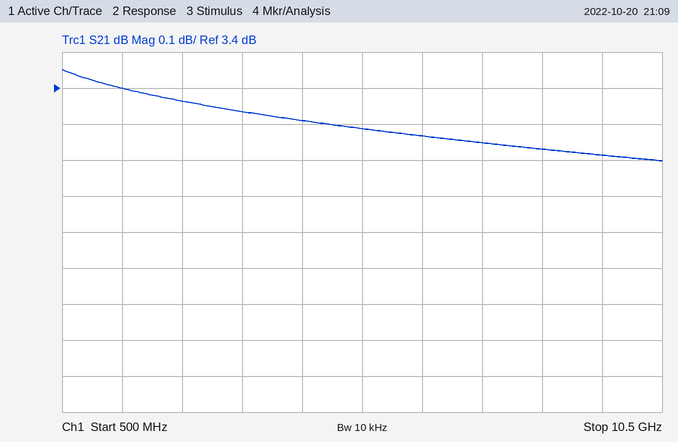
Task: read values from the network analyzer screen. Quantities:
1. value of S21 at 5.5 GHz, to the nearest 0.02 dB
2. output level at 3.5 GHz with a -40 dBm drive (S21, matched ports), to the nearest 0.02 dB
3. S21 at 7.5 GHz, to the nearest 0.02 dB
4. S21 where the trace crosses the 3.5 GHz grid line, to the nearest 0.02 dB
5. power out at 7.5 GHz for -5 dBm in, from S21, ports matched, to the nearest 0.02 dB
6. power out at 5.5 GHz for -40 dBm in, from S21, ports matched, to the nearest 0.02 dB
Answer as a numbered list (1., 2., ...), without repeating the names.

1. 3.28 dB
2. -36.66 dBm
3. 3.24 dB
4. 3.34 dB
5. -1.76 dBm
6. -36.72 dBm
